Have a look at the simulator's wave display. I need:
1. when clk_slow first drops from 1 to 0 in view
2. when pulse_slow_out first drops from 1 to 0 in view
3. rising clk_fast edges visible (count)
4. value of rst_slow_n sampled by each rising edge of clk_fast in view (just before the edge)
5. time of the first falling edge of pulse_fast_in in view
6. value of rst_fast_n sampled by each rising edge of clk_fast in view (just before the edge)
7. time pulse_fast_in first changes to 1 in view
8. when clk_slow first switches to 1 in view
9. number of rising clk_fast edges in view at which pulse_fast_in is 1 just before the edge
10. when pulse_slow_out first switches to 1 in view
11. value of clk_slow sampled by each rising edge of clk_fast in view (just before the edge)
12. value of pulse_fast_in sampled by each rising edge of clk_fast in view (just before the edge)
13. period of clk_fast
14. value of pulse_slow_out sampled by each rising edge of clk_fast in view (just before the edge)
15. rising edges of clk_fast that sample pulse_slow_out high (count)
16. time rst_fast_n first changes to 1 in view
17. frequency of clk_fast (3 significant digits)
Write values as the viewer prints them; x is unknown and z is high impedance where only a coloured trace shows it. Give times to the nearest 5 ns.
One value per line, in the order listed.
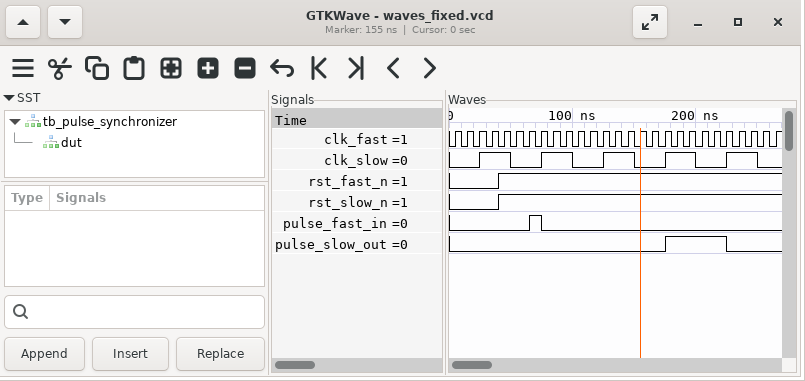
50 ns
225 ns
27
0 0 0 0 1 1 1 1 1 1 1 1 1 1 1 1 1 1 1 1 1 1 1 1 1 1 1
75 ns
0 0 0 0 1 1 1 1 1 1 1 1 1 1 1 1 1 1 1 1 1 1 1 1 1 1 1
65 ns
25 ns
1
175 ns
0 0 0 1 1 0 0 0 1 1 0 0 0 1 1 0 0 0 1 1 0 0 0 1 1 0 0
0 0 0 0 0 0 0 1 0 0 0 0 0 0 0 0 0 0 0 0 0 0 0 0 0 0 0
10 ns
0 0 0 0 0 0 0 0 0 0 0 0 0 0 0 0 0 0 1 1 1 1 1 0 0 0 0
5
40 ns
100 MHz
